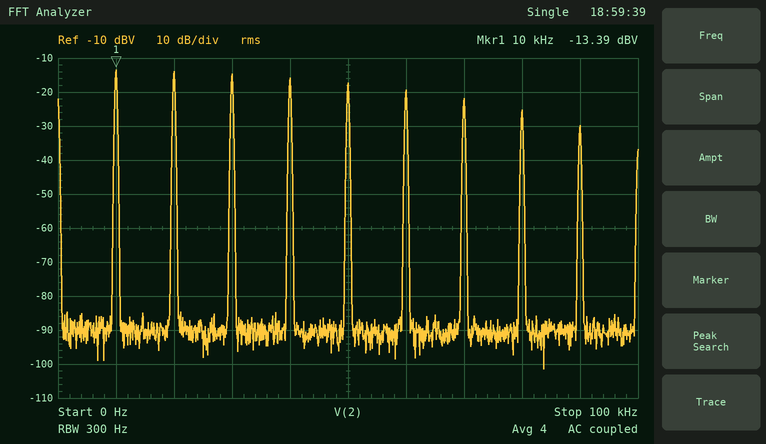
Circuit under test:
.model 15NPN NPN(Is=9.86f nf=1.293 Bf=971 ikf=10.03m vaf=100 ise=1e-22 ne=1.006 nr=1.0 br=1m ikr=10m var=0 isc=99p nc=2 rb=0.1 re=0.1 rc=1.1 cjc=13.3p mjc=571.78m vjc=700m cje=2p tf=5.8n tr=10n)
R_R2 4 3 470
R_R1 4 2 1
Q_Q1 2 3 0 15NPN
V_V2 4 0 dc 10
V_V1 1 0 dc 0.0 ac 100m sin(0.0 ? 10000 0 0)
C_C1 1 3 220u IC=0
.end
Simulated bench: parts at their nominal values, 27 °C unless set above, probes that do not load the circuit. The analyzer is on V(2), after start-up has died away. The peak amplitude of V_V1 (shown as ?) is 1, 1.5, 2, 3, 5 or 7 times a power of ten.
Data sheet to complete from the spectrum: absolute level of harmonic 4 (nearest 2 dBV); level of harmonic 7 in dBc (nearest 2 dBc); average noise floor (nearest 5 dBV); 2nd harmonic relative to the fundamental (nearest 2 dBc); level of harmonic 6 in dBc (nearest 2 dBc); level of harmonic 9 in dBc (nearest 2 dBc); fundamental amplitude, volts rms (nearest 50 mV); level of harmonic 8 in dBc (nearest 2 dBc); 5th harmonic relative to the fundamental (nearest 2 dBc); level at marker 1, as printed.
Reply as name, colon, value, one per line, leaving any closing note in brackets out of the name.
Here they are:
absolute level of harmonic 4: -16 dBV
level of harmonic 7 in dBc: -8 dBc
average noise floor: -90 dBV
2nd harmonic relative to the fundamental: 0 dBc
level of harmonic 6 in dBc: -6 dBc
level of harmonic 9 in dBc: -16 dBc
fundamental amplitude, volts rms: 200 mV
level of harmonic 8 in dBc: -12 dBc
5th harmonic relative to the fundamental: -4 dBc
level at marker 1, as printed: -13.39 dBV
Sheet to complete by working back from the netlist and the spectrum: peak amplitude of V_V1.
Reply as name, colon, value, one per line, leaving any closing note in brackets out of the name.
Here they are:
peak amplitude of V_V1: 5 V
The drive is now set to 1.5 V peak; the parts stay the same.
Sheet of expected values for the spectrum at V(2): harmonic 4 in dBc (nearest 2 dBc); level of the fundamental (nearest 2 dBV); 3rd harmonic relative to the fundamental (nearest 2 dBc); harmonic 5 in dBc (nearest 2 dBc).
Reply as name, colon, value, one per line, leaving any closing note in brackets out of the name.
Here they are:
harmonic 4 in dBc: -6 dBc
level of the fundamental: -12 dBV
3rd harmonic relative to the fundamental: -4 dBc
harmonic 5 in dBc: -12 dBc
